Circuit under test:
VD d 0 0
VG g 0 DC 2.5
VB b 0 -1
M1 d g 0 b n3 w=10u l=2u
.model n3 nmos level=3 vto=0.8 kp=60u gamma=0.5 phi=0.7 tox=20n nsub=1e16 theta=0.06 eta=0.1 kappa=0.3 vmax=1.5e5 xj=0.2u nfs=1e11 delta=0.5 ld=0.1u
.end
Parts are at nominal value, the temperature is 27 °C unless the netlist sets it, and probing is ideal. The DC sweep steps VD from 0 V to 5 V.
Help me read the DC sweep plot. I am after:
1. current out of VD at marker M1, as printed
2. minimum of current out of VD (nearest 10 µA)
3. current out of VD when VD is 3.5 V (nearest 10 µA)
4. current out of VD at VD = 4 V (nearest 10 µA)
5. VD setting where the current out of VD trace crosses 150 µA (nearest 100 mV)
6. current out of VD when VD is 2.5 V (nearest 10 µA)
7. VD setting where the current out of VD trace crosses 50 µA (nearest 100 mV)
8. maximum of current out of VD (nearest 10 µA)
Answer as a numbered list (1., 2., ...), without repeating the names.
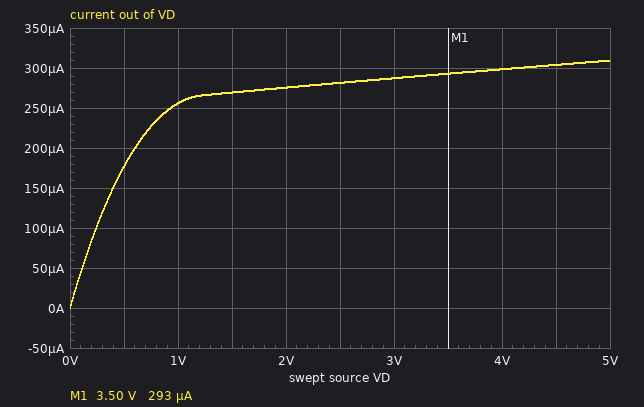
1. 293 µA
2. 0 A
3. 290 µA
4. 300 µA
5. 400 mV
6. 280 µA
7. 100 mV
8. 310 µA
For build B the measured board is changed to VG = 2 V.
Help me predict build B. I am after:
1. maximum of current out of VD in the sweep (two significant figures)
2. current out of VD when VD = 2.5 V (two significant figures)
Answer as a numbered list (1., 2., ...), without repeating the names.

1. 160 µA
2. 140 µA
